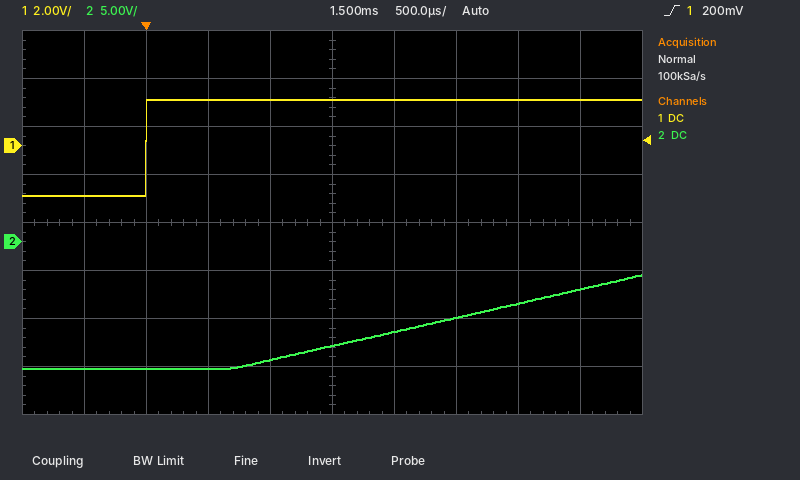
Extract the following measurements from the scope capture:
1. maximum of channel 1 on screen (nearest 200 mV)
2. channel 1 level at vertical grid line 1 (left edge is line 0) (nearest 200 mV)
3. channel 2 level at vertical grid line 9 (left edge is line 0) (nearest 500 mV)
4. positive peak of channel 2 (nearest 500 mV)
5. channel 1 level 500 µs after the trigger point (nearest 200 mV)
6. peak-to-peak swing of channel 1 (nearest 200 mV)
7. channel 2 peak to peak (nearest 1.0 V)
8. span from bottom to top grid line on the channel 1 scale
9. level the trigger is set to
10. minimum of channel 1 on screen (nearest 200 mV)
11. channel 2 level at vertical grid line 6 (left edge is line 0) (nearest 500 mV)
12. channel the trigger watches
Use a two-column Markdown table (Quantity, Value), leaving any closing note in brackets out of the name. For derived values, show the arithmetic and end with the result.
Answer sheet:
| Quantity | Value |
|---|---|
| maximum of channel 1 on screen | 2.0 V |
| channel 1 level at vertical grid line 1 (left edge is line 0) | -2.0 V |
| channel 2 level at vertical grid line 9 (left edge is line 0) | -5.0 V |
| positive peak of channel 2 | -3.5 V |
| channel 1 level 500 µs after the trigger point | 2.0 V |
| peak-to-peak swing of channel 1 | 2.0 V − (-2.0 V) = 4.0 V |
| channel 2 peak to peak | 10.0 V |
| span from bottom to top grid line on the channel 1 scale | 16 V |
| level the trigger is set to | 200 mV |
| minimum of channel 1 on screen | -2.0 V |
| channel 2 level at vertical grid line 6 (left edge is line 0) | -9.5 V |
| channel the trigger watches | channel 1 |
